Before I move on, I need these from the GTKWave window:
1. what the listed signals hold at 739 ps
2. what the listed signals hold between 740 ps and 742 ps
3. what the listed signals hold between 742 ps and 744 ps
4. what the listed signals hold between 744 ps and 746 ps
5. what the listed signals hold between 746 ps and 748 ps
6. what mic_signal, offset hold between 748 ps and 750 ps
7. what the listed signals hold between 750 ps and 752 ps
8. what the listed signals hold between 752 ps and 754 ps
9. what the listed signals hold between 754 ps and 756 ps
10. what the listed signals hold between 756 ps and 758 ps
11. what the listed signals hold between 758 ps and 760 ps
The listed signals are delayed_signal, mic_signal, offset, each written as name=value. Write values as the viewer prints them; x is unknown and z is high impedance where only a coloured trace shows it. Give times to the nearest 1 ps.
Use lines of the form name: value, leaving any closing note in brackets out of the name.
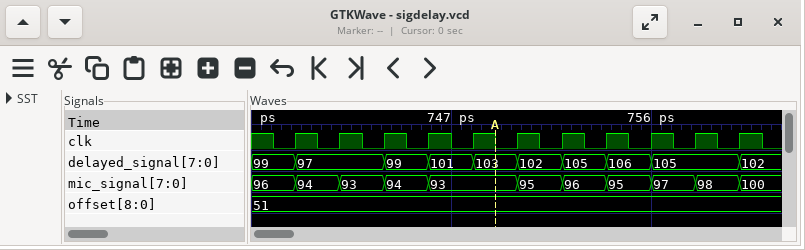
what the listed signals hold at 739 ps: delayed_signal=99, mic_signal=96, offset=51
what the listed signals hold between 740 ps and 742 ps: delayed_signal=97, mic_signal=94, offset=51
what the listed signals hold between 742 ps and 744 ps: delayed_signal=97, mic_signal=93, offset=51
what the listed signals hold between 744 ps and 746 ps: delayed_signal=99, mic_signal=94, offset=51
what the listed signals hold between 746 ps and 748 ps: delayed_signal=101, mic_signal=93, offset=51
what mic_signal, offset hold between 748 ps and 750 ps: mic_signal=93, offset=51
what the listed signals hold between 750 ps and 752 ps: delayed_signal=102, mic_signal=95, offset=51
what the listed signals hold between 752 ps and 754 ps: delayed_signal=105, mic_signal=96, offset=51
what the listed signals hold between 754 ps and 756 ps: delayed_signal=106, mic_signal=95, offset=51
what the listed signals hold between 756 ps and 758 ps: delayed_signal=105, mic_signal=97, offset=51
what the listed signals hold between 758 ps and 760 ps: delayed_signal=105, mic_signal=98, offset=51
